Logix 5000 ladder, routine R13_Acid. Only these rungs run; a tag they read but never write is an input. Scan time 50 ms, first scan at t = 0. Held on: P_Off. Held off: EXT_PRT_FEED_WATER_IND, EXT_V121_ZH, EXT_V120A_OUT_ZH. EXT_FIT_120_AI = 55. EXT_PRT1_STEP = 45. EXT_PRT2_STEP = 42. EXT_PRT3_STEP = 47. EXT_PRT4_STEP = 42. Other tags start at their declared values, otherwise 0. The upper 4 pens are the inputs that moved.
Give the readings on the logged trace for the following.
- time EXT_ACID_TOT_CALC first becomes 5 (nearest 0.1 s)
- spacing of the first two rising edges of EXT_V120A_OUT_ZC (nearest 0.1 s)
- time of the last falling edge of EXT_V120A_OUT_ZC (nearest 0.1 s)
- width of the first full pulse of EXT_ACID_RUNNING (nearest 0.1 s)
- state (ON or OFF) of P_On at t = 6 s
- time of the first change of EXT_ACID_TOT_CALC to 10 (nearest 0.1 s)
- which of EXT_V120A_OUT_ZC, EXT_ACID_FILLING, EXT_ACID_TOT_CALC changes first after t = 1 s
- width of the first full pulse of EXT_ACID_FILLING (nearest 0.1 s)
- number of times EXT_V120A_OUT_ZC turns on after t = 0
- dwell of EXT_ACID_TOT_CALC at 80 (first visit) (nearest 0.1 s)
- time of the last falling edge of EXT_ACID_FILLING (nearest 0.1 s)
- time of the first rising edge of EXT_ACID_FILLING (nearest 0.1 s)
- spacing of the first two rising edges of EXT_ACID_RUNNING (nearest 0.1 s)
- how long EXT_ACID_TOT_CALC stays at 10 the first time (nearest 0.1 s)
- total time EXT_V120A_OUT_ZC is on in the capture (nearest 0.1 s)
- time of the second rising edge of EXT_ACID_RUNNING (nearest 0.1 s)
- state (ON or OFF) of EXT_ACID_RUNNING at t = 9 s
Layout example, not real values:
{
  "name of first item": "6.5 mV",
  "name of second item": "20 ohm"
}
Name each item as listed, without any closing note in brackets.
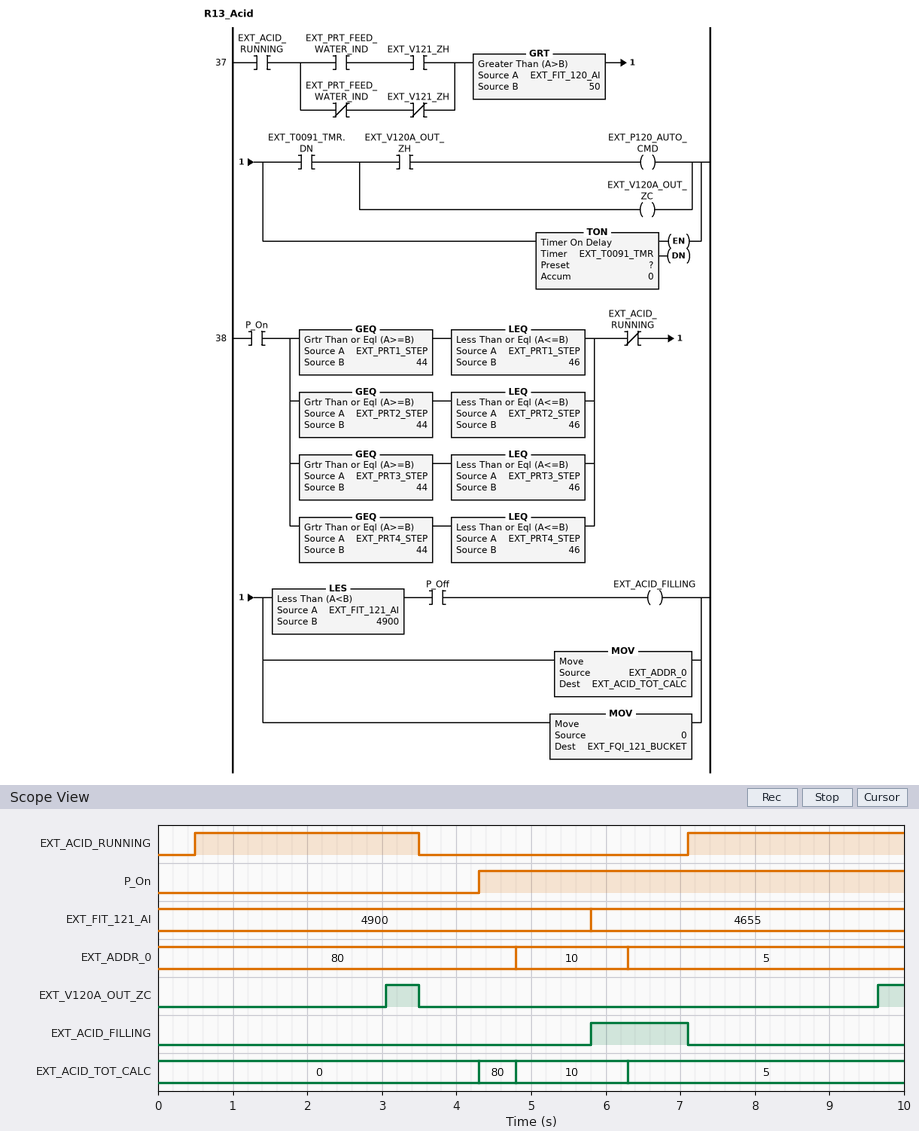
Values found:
{
  "time EXT_ACID_TOT_CALC first becomes 5": "6.3 s",
  "spacing of the first two rising edges of EXT_V120A_OUT_ZC": "6.6 s",
  "time of the last falling edge of EXT_V120A_OUT_ZC": "3.5 s",
  "width of the first full pulse of EXT_ACID_RUNNING": "3.0 s",
  "state (ON or OFF) of P_On at t = 6 s": "ON",
  "time of the first change of EXT_ACID_TOT_CALC to 10": "4.8 s",
  "which of EXT_V120A_OUT_ZC, EXT_ACID_FILLING, EXT_ACID_TOT_CALC changes first after t = 1 s": "EXT_V120A_OUT_ZC",
  "width of the first full pulse of EXT_ACID_FILLING": "1.3 s",
  "number of times EXT_V120A_OUT_ZC turns on after t = 0": "2",
  "dwell of EXT_ACID_TOT_CALC at 80 (first visit)": "0.5 s",
  "time of the last falling edge of EXT_ACID_FILLING": "7.1 s",
  "time of the first rising edge of EXT_ACID_FILLING": "5.8 s",
  "spacing of the first two rising edges of EXT_ACID_RUNNING": "6.6 s",
  "how long EXT_ACID_TOT_CALC stays at 10 the first time": "1.5 s",
  "total time EXT_V120A_OUT_ZC is on in the capture": "0.8 s",
  "time of the second rising edge of EXT_ACID_RUNNING": "7.1 s",
  "state (ON or OFF) of EXT_ACID_RUNNING at t = 9 s": "ON"
}
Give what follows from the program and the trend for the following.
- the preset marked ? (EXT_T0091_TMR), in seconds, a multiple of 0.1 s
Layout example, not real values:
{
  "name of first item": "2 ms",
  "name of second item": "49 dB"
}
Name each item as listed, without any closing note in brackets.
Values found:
{
  "the preset marked ? (EXT_T0091_TMR), in seconds, a multiple of 0.1 s": "2.5 s"
}
